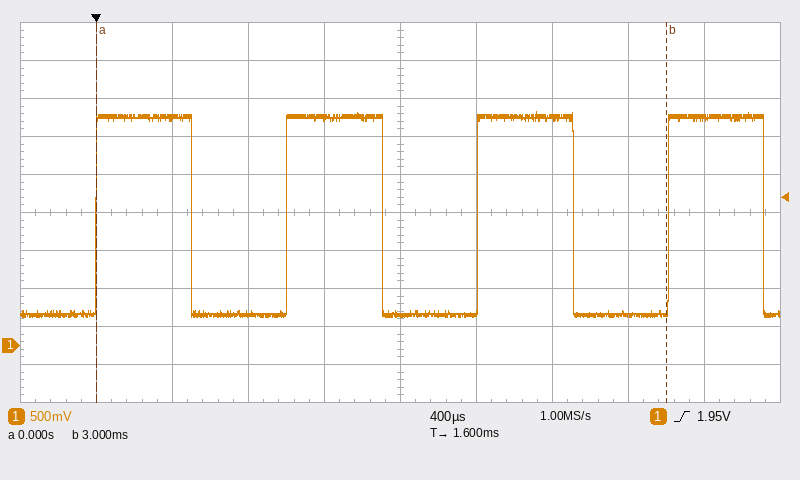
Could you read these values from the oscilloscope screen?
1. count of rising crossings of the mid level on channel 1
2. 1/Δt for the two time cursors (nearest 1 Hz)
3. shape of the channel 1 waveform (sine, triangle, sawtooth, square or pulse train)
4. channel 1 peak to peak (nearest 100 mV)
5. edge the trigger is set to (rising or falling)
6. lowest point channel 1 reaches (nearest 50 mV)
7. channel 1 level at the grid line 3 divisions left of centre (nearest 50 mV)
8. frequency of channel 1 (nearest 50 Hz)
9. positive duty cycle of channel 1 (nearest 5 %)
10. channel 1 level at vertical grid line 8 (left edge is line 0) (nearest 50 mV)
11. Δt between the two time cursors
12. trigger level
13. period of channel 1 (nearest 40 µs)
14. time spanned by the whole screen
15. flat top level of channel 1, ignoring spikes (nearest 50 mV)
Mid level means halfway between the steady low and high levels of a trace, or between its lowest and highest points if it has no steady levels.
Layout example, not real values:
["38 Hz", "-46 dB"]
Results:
["4", "333 Hz", "square", "2.70 V", "rising", "400 mV", "3.00 V", "1.00 kHz", "50 %", "400 mV", "3.00 ms", "1.95 V", "1.00 ms", "4 ms", "3.00 V"]
